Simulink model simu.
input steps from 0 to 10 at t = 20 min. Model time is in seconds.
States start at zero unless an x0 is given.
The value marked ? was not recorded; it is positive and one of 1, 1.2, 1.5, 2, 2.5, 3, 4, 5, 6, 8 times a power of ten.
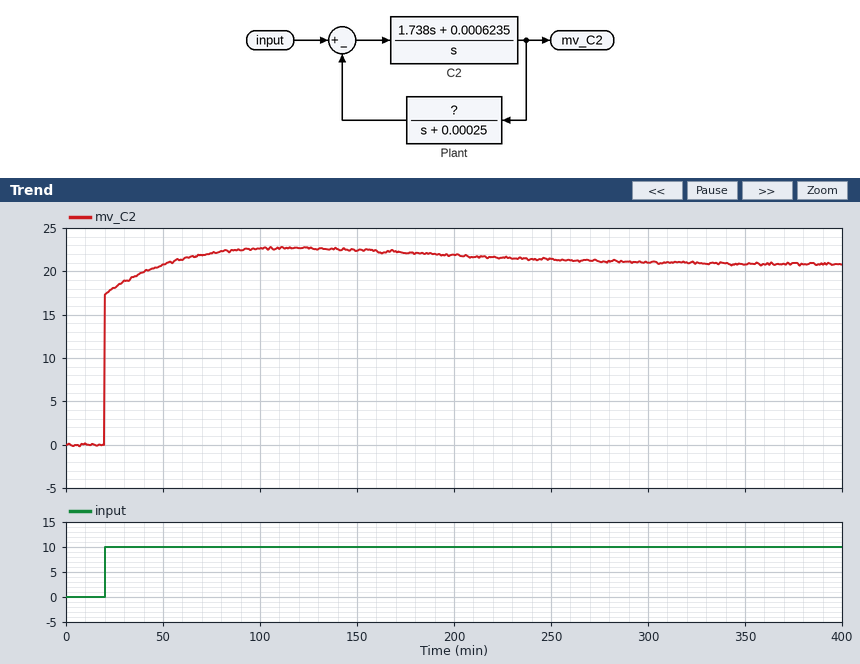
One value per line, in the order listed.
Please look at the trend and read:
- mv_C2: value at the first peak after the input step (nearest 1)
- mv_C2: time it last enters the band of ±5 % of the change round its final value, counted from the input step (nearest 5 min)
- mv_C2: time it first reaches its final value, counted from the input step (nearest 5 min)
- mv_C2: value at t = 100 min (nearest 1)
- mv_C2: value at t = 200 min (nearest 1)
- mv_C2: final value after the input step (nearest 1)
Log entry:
23
180 min
30 min
23
22
21
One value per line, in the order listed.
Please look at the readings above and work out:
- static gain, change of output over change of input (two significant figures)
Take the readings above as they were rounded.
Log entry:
2.1
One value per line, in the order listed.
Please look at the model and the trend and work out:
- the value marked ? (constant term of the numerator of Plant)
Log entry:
0.00012
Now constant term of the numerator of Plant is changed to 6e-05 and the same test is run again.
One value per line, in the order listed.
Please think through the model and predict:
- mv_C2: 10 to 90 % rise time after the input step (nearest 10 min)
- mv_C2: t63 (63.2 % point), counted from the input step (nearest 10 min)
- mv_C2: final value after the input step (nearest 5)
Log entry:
140 min
40 min
40
